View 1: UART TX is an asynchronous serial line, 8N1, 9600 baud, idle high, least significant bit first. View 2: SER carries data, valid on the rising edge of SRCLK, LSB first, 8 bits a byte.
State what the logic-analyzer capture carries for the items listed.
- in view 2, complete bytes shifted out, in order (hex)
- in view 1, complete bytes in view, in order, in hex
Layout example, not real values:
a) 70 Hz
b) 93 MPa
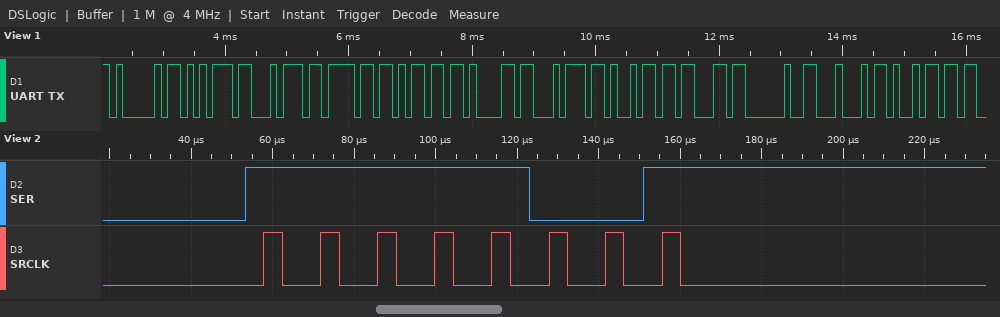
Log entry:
a) 0x9F
b) 41 75 74 6F 6D 61 74 69 63 20 44 69
